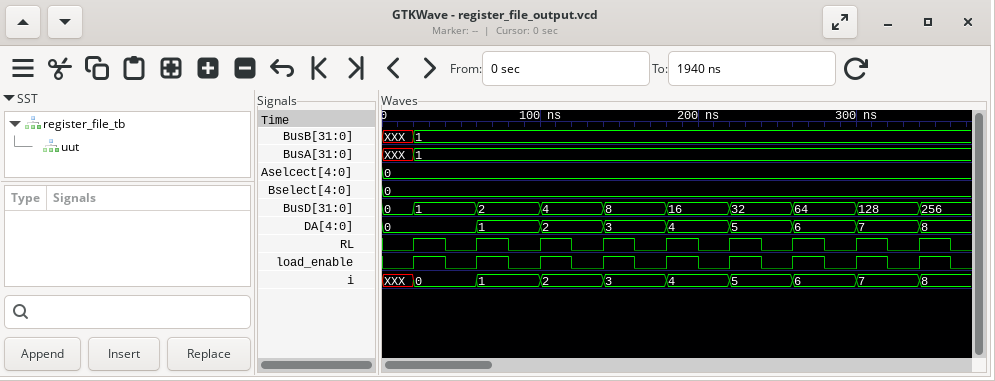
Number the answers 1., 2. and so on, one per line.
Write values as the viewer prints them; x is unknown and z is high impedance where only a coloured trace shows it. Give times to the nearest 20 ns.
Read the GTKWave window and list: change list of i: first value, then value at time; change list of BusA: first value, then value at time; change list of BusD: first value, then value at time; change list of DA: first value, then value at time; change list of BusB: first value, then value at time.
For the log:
1. XXX, 0 at 20 ns, 1 at 60 ns, 2 at 100 ns, 3 at 140 ns, 4 at 180 ns, 5 at 220 ns, 6 at 260 ns, 7 at 300 ns, 8 at 340 ns
2. XXX, 1 at 20 ns
3. 0, 1 at 20 ns, 2 at 60 ns, 4 at 100 ns, 8 at 140 ns, 16 at 180 ns, 32 at 220 ns, 64 at 260 ns, 128 at 300 ns, 256 at 340 ns
4. 0, 1 at 60 ns, 2 at 100 ns, 3 at 140 ns, 4 at 180 ns, 5 at 220 ns, 6 at 260 ns, 7 at 300 ns, 8 at 340 ns
5. XXX, 1 at 20 ns
